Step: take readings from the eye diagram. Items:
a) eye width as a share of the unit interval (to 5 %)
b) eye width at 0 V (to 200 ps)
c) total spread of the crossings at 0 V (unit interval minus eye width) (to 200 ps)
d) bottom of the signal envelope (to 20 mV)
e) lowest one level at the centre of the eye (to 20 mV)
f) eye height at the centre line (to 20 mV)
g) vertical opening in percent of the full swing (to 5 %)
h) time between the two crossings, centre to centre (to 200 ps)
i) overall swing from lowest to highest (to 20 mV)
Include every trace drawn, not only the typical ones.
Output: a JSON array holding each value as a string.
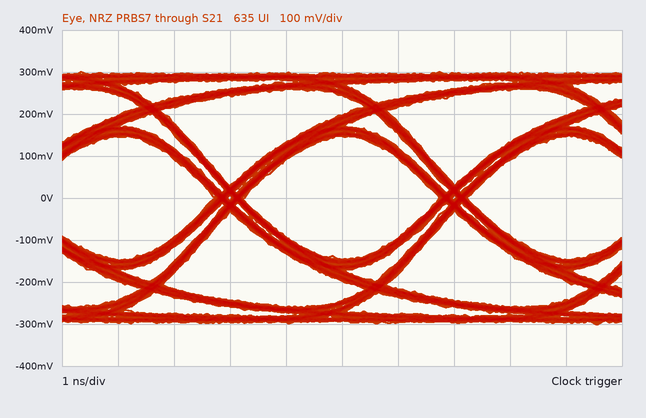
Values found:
["85 %", "3.4 ns", "600 ps", "-300 mV", "140 mV", "300 mV", "50 %", "4.0 ns", "600 mV"]
